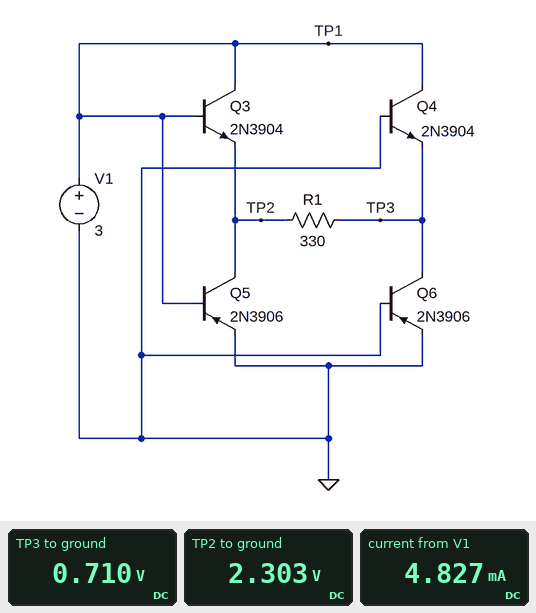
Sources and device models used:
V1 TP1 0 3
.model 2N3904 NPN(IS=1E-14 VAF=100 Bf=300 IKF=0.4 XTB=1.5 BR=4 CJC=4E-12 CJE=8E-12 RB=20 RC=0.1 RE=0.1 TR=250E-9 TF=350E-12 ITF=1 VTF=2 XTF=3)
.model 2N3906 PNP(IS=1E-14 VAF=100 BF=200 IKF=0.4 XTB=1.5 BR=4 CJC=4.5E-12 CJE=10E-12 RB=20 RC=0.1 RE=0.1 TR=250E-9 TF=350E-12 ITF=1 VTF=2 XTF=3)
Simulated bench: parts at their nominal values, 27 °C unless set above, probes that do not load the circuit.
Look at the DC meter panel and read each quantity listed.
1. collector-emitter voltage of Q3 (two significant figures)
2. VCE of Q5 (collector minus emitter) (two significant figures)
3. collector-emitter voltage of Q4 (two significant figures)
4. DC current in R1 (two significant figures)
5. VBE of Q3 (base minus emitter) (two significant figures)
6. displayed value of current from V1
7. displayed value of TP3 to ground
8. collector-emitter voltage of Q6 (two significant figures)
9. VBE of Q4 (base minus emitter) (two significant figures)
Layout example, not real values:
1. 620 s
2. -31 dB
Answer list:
1. 700 mV
2. 2.3 V
3. 2.3 V
4. 4.8 mA
5. 700 mV
6. 4.827 mA
7. 0.710 V
8. 710 mV
9. -710 mV
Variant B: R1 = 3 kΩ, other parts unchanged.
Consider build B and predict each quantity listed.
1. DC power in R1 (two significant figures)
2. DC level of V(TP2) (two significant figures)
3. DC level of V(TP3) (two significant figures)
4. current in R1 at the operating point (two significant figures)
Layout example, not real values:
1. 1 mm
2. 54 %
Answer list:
1. 990 µW
2. 2.4 V
3. 640 mV
4. 570 µA
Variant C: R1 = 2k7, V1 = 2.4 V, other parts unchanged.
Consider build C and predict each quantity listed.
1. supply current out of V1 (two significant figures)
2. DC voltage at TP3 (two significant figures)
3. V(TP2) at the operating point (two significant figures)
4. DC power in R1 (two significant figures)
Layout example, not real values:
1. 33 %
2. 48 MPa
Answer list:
1. 420 µA
2. 630 mV
3. 1.8 V
4. 480 µW
